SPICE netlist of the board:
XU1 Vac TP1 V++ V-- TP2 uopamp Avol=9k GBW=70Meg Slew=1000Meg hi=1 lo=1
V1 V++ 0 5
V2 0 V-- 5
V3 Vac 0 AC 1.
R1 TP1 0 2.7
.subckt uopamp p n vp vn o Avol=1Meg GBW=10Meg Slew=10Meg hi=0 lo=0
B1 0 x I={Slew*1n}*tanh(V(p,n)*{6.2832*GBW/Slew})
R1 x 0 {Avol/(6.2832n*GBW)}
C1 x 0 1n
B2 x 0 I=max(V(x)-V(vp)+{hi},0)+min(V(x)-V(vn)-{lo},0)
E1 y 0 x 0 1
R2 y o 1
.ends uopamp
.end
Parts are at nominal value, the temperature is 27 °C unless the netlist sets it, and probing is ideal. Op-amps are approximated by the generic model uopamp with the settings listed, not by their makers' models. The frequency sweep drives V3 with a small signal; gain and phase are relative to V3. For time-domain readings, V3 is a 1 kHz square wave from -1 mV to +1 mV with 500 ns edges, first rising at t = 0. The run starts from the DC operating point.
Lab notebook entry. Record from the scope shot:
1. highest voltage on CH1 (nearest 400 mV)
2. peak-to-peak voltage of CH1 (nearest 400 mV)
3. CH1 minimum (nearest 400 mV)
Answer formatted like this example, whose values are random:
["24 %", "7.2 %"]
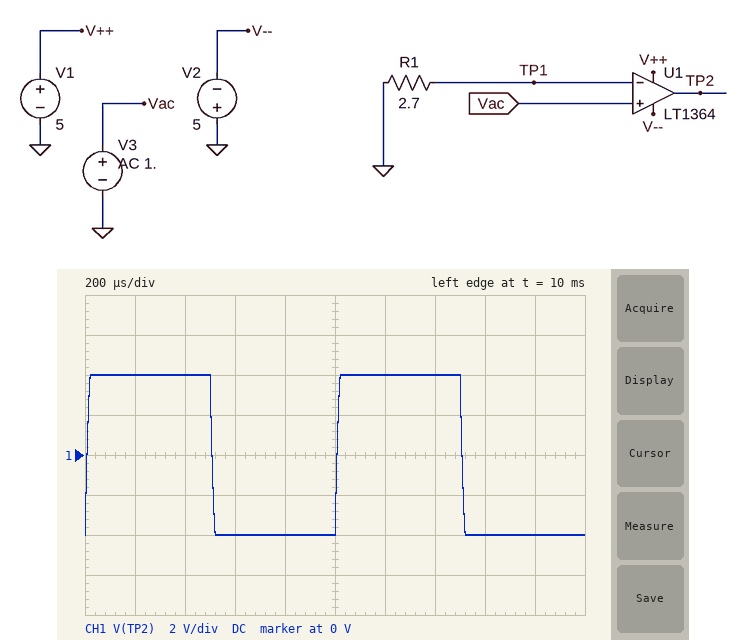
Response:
["4.0 V", "8.0 V", "-4.0 V"]
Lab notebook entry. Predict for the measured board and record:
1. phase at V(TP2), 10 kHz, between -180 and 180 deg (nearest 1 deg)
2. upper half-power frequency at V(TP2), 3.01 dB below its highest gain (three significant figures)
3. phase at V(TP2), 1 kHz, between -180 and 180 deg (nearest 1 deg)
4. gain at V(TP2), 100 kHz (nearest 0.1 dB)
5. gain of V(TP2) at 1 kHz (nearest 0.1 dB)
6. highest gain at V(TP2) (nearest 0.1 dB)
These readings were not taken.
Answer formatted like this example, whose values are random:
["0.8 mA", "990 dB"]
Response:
["-52 deg", "7.78 kHz", "-7 deg", "56.9 dB", "79.0 dB", "79.1 dB"]
